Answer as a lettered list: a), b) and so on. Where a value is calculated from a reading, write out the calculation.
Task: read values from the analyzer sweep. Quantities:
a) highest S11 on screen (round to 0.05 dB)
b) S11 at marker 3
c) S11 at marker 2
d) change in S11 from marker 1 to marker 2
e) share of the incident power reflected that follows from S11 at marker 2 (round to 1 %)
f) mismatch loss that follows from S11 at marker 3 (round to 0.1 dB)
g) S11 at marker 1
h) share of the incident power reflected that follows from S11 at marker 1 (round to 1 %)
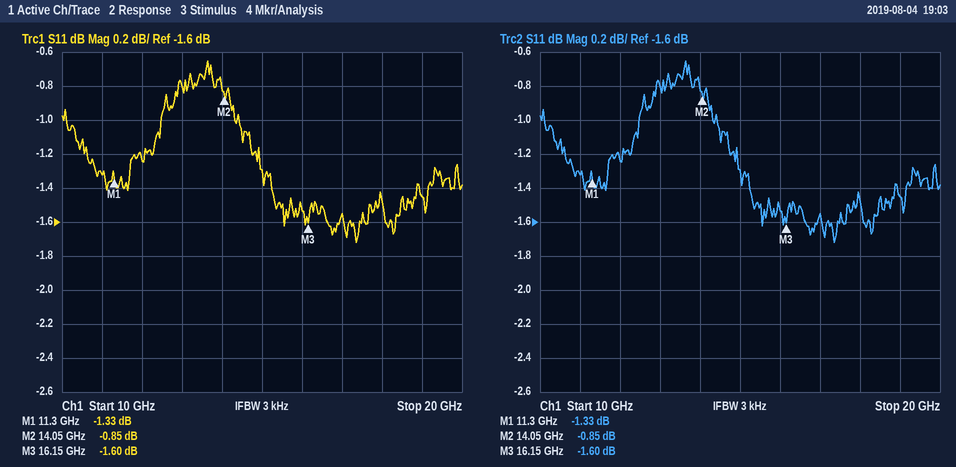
a) -0.65 dB
b) -1.60 dB
c) -0.85 dB
d) -0.85 − (-1.33) = 0.48 dB
e) 10^(-0.85/10) ≈ 82 %
f) −10 log10(1 − 10^(-1.6/10)) ≈ 5.1 dB
g) -1.33 dB
h) 10^(-1.33/10) ≈ 74 %
